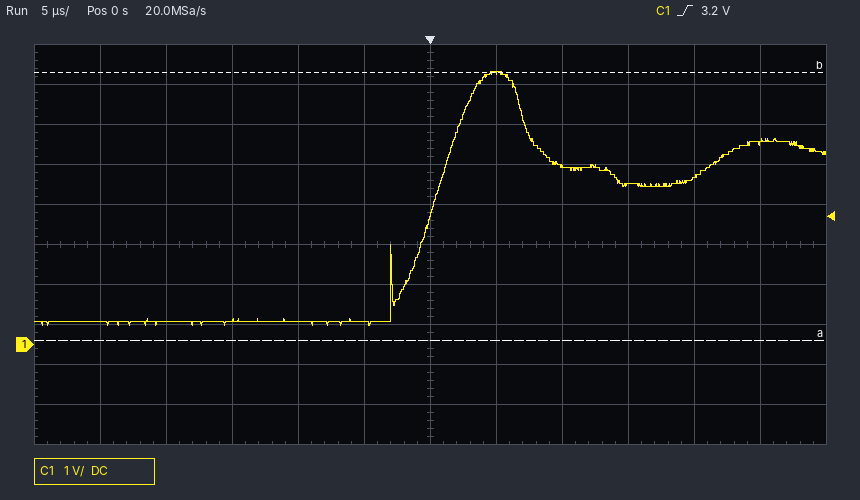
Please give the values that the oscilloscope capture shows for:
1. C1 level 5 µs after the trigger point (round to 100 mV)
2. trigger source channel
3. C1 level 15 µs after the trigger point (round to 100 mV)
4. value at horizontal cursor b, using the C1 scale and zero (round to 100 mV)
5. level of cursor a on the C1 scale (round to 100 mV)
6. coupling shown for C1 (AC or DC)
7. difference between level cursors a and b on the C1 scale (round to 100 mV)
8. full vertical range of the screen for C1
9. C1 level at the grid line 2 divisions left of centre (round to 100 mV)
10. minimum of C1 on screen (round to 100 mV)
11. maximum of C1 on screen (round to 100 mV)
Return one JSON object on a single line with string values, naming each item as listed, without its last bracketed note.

{"C1 level 5 µs after the trigger point": "6.8 V", "trigger source channel": "C1", "C1 level 15 µs after the trigger point": "4.0 V", "value at horizontal cursor b, using the C1 scale and zero": "6.8 V", "level of cursor a on the C1 scale": "100 mV", "coupling shown for C1": "DC", "difference between level cursors a and b on the C1 scale": "6.7 V", "full vertical range of the screen for C1": "10 V", "C1 level at the grid line 2 divisions left of centre": "600 mV", "minimum of C1 on screen": "500 mV", "maximum of C1 on screen": "6.8 V"}
